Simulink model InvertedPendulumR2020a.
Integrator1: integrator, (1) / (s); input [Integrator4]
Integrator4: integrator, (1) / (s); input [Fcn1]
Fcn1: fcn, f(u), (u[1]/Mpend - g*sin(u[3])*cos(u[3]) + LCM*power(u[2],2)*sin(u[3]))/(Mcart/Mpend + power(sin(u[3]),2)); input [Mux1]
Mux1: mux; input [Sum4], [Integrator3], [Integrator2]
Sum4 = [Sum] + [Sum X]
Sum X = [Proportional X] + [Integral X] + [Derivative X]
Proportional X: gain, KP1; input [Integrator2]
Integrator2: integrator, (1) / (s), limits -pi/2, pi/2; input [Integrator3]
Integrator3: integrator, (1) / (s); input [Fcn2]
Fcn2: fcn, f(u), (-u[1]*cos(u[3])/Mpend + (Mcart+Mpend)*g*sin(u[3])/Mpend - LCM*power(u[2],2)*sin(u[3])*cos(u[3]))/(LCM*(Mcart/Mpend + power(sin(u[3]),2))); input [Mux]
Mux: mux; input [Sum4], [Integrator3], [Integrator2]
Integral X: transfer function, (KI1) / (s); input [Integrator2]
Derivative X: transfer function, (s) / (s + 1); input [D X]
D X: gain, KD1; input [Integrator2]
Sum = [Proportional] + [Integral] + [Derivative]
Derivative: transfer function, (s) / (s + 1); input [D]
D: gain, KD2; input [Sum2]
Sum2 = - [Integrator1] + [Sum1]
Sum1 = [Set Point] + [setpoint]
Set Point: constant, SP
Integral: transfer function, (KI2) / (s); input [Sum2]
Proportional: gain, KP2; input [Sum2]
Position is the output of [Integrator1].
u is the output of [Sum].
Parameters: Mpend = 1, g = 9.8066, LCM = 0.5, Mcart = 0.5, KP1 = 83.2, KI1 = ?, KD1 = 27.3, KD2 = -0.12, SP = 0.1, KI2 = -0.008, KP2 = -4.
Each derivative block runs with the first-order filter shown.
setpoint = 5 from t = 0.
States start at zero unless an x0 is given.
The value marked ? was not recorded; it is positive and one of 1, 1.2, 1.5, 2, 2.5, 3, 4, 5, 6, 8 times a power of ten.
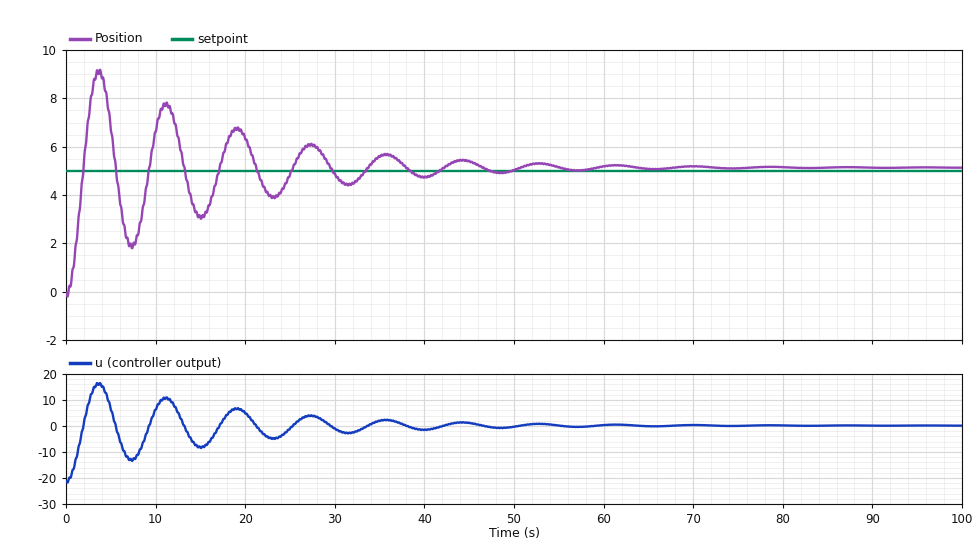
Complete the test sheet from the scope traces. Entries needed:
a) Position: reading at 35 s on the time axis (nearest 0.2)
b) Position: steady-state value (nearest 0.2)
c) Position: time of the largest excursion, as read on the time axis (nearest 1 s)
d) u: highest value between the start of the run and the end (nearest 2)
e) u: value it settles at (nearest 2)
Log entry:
5.6
5.2
4 s
16
0
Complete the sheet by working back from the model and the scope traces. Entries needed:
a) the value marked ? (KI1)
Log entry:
20
